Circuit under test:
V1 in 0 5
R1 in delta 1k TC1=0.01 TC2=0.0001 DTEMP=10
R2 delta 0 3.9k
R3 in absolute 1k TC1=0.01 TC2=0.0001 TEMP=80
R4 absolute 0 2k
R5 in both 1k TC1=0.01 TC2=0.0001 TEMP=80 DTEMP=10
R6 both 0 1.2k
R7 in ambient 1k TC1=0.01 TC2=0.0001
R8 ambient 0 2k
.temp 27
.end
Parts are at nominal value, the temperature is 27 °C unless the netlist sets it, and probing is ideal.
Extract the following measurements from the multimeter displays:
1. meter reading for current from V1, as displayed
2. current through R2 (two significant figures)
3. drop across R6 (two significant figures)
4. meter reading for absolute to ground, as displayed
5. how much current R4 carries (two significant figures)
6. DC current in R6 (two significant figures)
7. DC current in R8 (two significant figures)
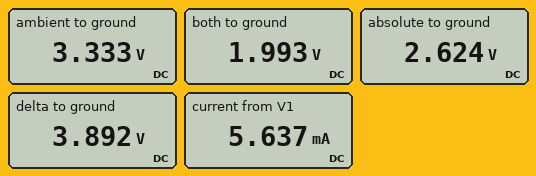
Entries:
5.637 mA
1.0 mA
2.0 V
2.624 V
1.3 mA
1.7 mA
1.7 mA
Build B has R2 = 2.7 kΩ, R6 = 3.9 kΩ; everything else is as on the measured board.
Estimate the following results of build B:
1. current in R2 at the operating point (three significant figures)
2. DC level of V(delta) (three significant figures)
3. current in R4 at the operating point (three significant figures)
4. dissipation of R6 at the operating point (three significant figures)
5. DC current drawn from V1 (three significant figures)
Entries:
1.31 mA
3.54 V
1.31 mA
2.99 mW
5.17 mA
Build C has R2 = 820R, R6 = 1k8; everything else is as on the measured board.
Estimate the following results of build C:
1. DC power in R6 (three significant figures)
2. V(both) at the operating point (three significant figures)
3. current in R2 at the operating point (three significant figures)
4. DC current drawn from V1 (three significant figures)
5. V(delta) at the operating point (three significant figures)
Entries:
3.45 mW
2.49 V
2.59 mA
6.95 mA
2.12 V
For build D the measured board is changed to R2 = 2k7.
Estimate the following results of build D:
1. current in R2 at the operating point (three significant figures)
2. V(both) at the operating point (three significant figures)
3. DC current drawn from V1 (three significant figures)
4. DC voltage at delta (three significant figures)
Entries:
1.31 mA
1.99 V
5.95 mA
3.54 V
